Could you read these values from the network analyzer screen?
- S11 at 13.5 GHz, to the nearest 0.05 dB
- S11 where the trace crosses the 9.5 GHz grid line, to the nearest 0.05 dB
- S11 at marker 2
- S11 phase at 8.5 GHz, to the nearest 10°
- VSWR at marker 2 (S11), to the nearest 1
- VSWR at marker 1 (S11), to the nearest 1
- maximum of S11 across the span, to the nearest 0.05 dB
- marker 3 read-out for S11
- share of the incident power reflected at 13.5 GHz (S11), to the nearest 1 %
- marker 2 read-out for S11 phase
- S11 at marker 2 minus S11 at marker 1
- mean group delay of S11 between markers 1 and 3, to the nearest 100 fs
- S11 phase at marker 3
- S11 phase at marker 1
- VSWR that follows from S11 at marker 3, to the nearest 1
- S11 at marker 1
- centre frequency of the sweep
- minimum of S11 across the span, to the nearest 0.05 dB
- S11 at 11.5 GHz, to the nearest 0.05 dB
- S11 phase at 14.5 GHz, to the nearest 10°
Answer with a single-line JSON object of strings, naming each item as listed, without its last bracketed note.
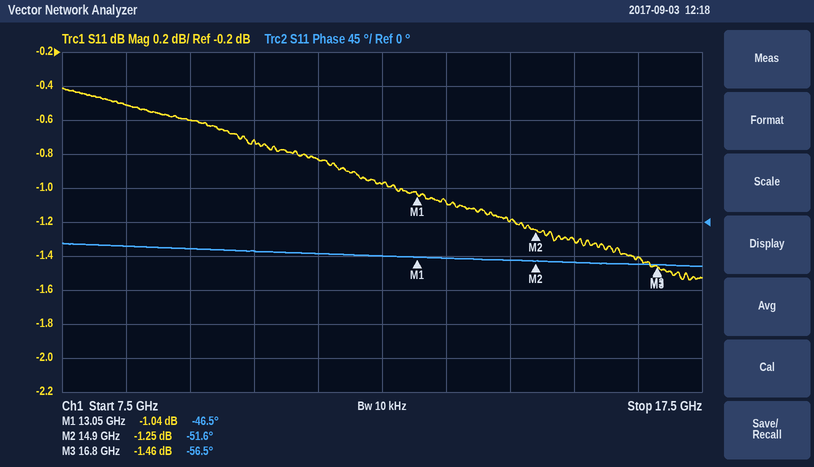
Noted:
{"S11 at 13.5 GHz, to the nearest 0.05 dB": "-1.10 dB", "S11 where the trace crosses the 9.5 GHz grid line, to the nearest 0.05 dB": "-0.60 dB", "S11 at marker 2": "-1.25 dB", "S11 phase at 8.5 GHz, to the nearest 10°": "-30°", "VSWR at marker 2 (S11), to the nearest 1": "14", "VSWR at marker 1 (S11), to the nearest 1": "17", "maximum of S11 across the span, to the nearest 0.05 dB": "-0.40 dB", "marker 3 read-out for S11": "-1.46 dB", "share of the incident power reflected at 13.5 GHz (S11), to the nearest 1 %": "78 %", "marker 2 read-out for S11 phase": "-51.6°", "S11 at marker 2 minus S11 at marker 1": "-0.21 dB", "mean group delay of S11 between markers 1 and 3, to the nearest 100 fs": "7.4 ps", "S11 phase at marker 3": "-56.5°", "S11 phase at marker 1": "-46.5°", "VSWR that follows from S11 at marker 3, to the nearest 1": "12", "S11 at marker 1": "-1.04 dB", "centre frequency of the sweep": "12.5 GHz", "minimum of S11 across the span, to the nearest 0.05 dB": "-1.55 dB", "S11 at 11.5 GHz, to the nearest 0.05 dB": "-0.85 dB", "S11 phase at 14.5 GHz, to the nearest 10°": "-50°"}
